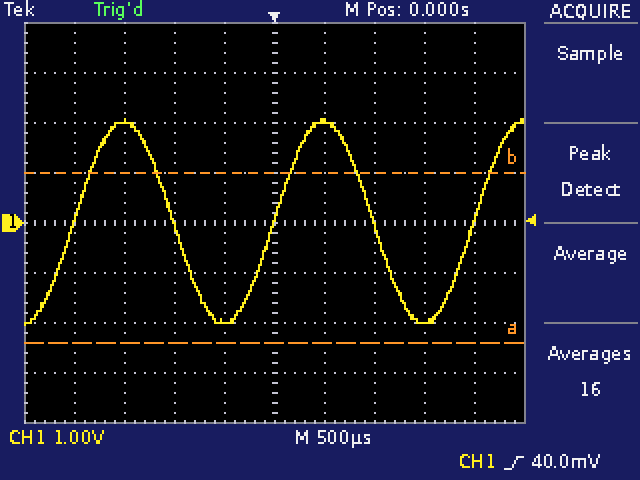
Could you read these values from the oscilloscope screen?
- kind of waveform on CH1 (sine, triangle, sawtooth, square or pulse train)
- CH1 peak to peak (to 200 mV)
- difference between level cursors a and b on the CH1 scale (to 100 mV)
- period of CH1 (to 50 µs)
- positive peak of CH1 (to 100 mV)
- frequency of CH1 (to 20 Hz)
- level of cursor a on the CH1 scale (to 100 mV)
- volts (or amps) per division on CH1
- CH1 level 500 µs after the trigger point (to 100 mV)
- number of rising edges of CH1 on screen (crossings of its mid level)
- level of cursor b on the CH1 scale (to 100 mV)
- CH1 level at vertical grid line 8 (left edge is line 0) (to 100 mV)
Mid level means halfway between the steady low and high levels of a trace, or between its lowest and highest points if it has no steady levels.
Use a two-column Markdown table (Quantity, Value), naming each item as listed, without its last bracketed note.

| Quantity | Value |
|---|---|
| kind of waveform on CH1 | sine |
| CH1 peak to peak | 4.2 V |
| difference between level cursors a and b on the CH1 scale | 3.4 V |
| period of CH1 | 2.00 ms |
| positive peak of CH1 | 2.1 V |
| frequency of CH1 | 500 Hz |
| level of cursor a on the CH1 scale | -2.4 V |
| volts (or amps) per division on CH1 | 1 V |
| CH1 level 500 µs after the trigger point | 2.0 V |
| number of rising edges of CH1 on screen | 3 |
| level of cursor b on the CH1 scale | 1.0 V |
| CH1 level at vertical grid line 8 (left edge is line 0) | -2.0 V |
